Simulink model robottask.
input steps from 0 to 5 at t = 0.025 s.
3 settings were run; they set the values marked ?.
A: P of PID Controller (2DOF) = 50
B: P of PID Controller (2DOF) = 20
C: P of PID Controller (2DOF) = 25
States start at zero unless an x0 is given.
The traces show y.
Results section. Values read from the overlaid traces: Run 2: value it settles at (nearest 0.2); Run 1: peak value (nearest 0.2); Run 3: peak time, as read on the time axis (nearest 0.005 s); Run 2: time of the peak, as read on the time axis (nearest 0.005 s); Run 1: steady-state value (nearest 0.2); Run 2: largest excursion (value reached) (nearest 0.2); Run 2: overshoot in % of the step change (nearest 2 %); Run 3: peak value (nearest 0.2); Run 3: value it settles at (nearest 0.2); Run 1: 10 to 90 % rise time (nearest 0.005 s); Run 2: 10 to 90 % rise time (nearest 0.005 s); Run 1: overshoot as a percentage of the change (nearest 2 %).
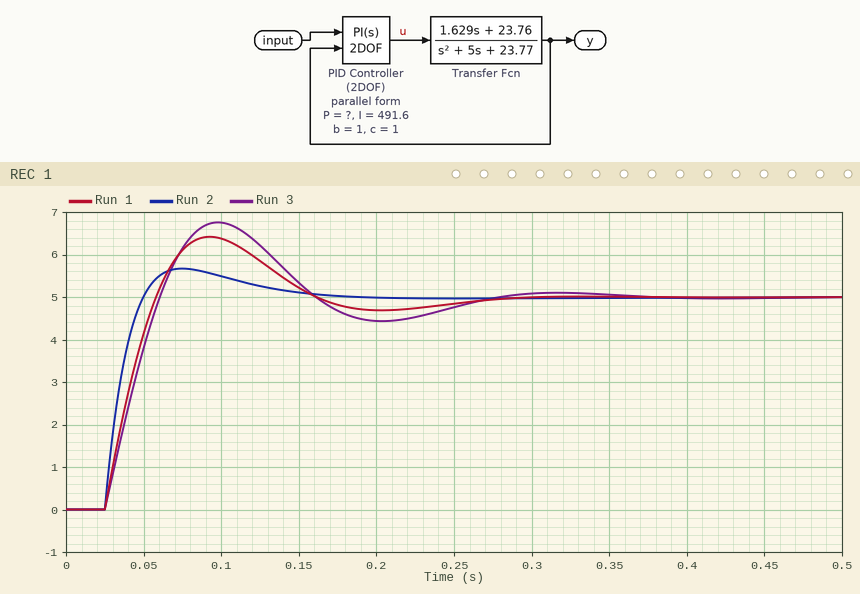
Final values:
5.0
6.4
0.100 s
0.075 s
5.0
5.6
14 %
6.8
5.0
0.025 s
0.020 s
28 %
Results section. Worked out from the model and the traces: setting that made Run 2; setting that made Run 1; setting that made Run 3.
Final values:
A
C
B
